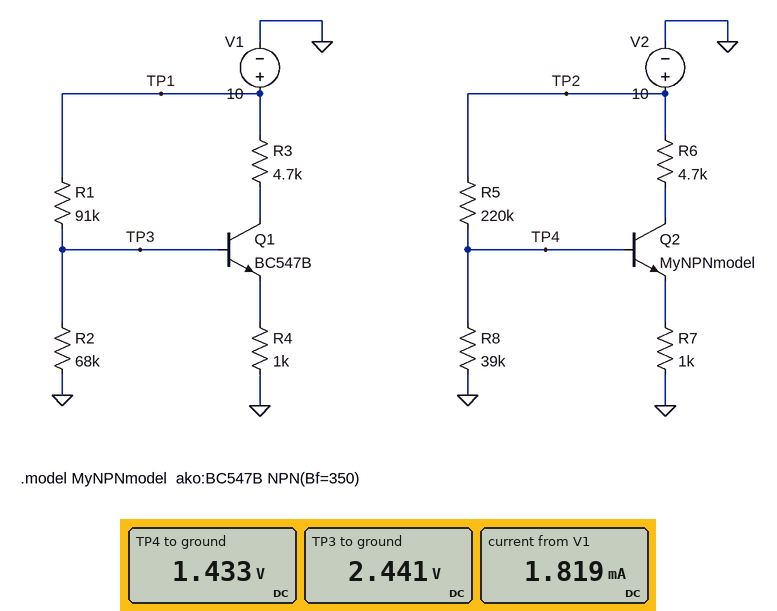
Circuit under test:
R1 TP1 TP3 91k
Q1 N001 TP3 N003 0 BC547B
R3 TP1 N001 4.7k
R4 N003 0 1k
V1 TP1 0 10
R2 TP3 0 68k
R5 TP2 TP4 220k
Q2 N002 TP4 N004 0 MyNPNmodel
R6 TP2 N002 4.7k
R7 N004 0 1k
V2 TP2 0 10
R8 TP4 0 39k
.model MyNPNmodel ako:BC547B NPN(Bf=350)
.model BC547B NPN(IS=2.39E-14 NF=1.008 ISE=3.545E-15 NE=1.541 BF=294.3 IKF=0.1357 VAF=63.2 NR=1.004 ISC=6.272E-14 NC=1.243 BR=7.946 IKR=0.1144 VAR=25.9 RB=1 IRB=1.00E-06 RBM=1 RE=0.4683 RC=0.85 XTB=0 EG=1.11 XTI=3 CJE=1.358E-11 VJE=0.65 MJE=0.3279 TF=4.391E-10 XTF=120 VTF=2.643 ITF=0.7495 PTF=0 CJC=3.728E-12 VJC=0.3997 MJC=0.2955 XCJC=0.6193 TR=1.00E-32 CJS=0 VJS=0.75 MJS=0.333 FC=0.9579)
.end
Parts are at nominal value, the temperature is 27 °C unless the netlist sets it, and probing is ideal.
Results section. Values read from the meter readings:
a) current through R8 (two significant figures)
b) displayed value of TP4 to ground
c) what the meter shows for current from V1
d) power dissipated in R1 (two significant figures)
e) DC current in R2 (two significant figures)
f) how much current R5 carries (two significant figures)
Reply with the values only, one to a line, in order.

37 µA
1.433 V
1.819 mA
630 µW
36 µA
39 µA
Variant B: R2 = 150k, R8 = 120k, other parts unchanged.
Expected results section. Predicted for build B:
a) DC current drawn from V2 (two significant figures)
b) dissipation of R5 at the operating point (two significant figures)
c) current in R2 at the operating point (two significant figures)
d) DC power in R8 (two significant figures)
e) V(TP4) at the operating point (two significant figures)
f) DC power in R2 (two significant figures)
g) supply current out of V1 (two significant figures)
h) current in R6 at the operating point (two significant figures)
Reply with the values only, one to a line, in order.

1.8 mA
260 µW
16 µA
48 µW
2.4 V
40 µW
1.8 mA
1.7 mA
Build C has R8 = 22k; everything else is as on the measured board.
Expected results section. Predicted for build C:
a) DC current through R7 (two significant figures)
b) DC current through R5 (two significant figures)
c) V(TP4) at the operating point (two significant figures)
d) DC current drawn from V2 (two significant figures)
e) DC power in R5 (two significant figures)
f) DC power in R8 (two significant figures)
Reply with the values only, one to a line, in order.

290 µA
41 µA
890 mV
330 µA
380 µW
36 µW
